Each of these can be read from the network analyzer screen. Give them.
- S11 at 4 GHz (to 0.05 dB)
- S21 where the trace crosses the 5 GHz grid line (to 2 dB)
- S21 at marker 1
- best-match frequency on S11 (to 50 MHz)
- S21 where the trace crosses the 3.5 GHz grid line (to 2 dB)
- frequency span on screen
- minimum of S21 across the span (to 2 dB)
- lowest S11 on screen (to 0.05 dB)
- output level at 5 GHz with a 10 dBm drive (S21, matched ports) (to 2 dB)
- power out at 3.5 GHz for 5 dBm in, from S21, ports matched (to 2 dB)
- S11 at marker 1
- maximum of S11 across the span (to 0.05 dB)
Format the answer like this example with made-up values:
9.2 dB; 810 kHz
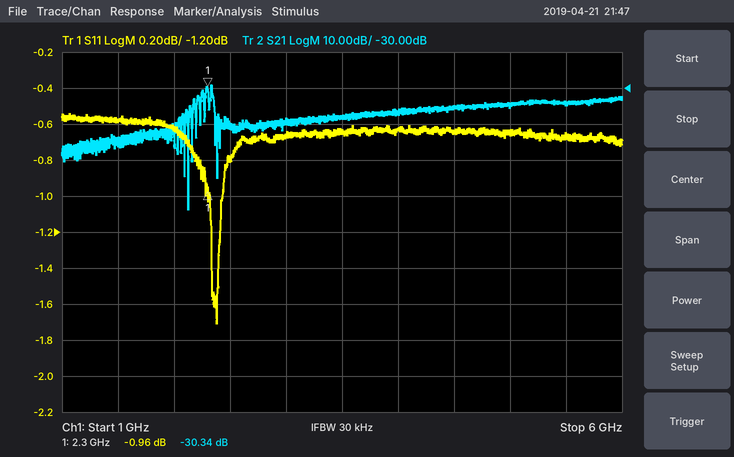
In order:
-0.65 dB; -34 dB; -30.34 dB; 2.40 GHz; -38 dB; 5 GHz; -64 dB; -1.70 dB; -24 dBm; -34 dBm; -0.96 dB; -0.55 dB
